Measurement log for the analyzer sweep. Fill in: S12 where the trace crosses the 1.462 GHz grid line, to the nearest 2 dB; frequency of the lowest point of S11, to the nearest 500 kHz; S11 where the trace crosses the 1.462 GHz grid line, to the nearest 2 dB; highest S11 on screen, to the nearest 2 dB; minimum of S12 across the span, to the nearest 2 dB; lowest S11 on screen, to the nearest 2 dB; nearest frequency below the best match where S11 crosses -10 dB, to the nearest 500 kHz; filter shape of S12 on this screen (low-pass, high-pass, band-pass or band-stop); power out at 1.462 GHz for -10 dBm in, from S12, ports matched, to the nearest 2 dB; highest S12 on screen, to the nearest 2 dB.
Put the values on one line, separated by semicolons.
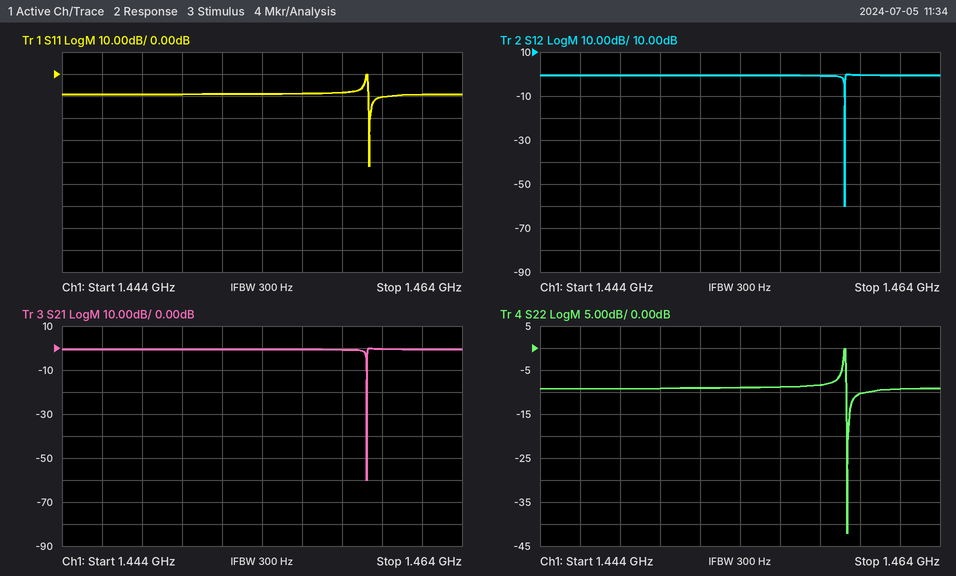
0 dB; 1.4595 GHz; -10 dB; 0 dB; -60 dB; -42 dB; 1.4595 GHz; band-stop; -10 dBm; 0 dB
